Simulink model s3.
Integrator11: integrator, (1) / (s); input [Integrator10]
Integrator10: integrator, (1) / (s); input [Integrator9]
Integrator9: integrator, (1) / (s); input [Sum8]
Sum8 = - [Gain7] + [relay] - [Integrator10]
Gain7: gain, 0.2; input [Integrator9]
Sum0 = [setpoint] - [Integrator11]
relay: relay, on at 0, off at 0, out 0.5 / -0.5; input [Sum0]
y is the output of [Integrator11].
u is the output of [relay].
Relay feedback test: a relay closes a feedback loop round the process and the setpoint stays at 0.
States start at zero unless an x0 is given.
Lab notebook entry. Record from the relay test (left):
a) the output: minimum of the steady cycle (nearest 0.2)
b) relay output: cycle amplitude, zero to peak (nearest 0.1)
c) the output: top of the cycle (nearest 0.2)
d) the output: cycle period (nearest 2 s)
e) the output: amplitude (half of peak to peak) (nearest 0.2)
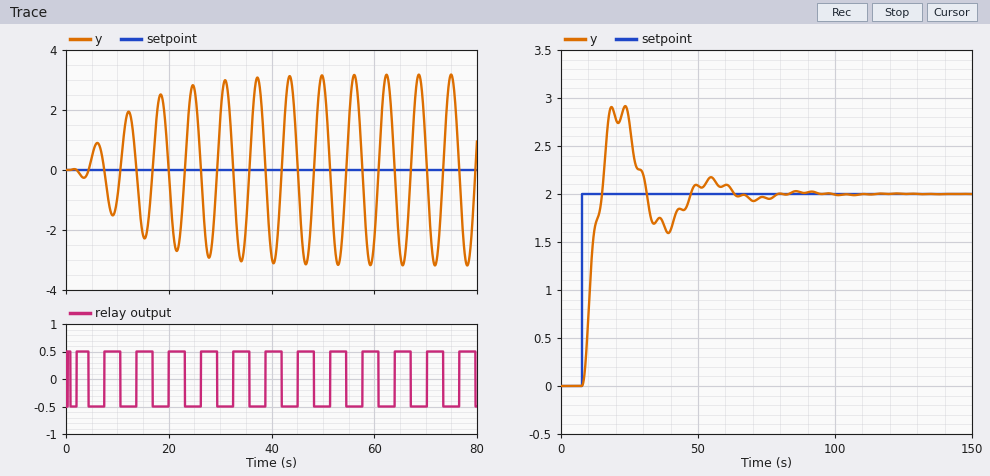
-3.2
0.5
3.2
6 s
3.2
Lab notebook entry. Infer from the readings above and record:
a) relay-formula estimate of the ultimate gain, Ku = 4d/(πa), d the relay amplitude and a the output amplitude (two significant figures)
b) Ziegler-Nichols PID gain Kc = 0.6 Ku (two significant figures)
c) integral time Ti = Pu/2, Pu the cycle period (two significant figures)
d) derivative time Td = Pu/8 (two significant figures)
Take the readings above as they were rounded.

0.20
0.12
3.0 s
0.75 s
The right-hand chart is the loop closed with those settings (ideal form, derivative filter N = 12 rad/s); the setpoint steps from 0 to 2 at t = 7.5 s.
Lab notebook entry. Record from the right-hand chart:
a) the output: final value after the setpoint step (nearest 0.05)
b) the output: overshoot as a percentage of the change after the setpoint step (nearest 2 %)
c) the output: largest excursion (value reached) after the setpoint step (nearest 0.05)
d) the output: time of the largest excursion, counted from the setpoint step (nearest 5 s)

2.00
46 %
2.90
15 s
